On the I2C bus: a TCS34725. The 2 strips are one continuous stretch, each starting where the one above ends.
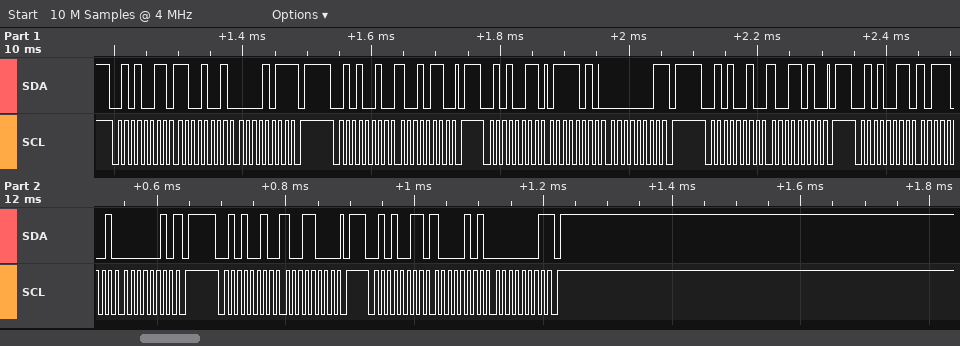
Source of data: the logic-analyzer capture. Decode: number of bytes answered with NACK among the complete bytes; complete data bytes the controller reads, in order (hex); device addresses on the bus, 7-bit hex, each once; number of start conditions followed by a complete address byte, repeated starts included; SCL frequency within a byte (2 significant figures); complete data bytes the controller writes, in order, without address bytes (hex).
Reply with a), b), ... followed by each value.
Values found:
a) 4
b) C9 0B 7A 01 B9 02 85 01
c) 0x29
d) 7
e) 100 kHz
f) 96 9A 98
